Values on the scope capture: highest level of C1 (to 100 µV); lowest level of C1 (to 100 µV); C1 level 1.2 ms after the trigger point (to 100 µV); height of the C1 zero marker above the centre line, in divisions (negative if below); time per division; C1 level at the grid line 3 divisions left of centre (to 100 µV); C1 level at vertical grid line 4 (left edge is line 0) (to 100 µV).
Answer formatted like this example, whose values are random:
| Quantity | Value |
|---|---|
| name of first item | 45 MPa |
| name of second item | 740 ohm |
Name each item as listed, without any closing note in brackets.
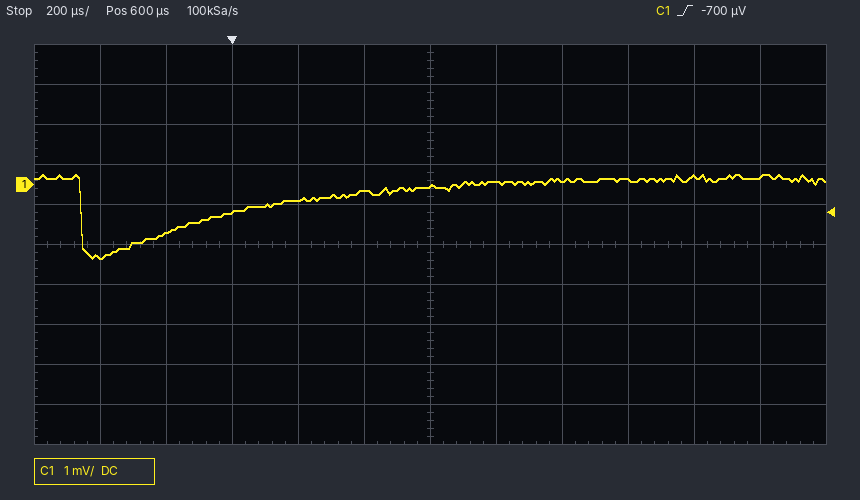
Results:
| Quantity | Value |
|---|---|
| highest level of C1 | 200 µV |
| lowest level of C1 | -1.8 mV |
| C1 level 1.2 ms after the trigger point | 100 µV |
| height of the C1 zero marker above the centre line, in divisions | +1.5 div |
| time per division | 200 µs |
| C1 level at the grid line 3 divisions left of centre | -700 µV |
| C1 level at vertical grid line 4 (left edge is line 0) | -400 µV |
